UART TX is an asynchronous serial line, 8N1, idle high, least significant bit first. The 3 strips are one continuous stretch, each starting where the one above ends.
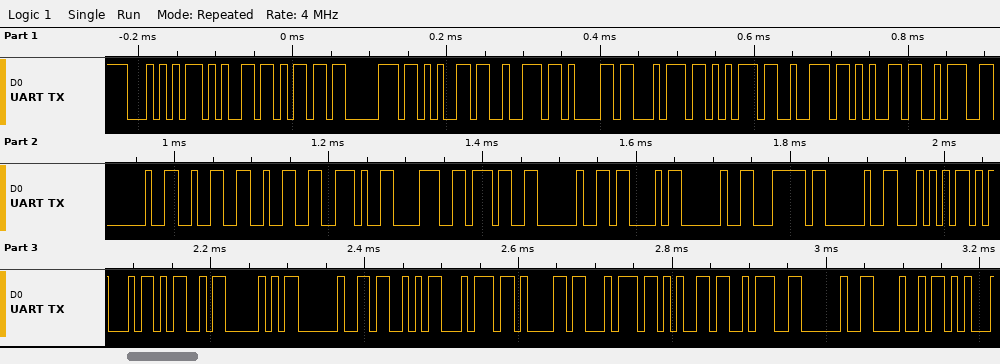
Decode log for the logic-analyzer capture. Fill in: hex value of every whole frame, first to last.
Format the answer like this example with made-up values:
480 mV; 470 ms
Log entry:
54 65 6D 70 65 72 61 74 75 72 65 3A 20 32 32 2E 38 37 20 43 20 7C 20 54 45 4D 50 20 53 74 61 74 65 3A 20 48
